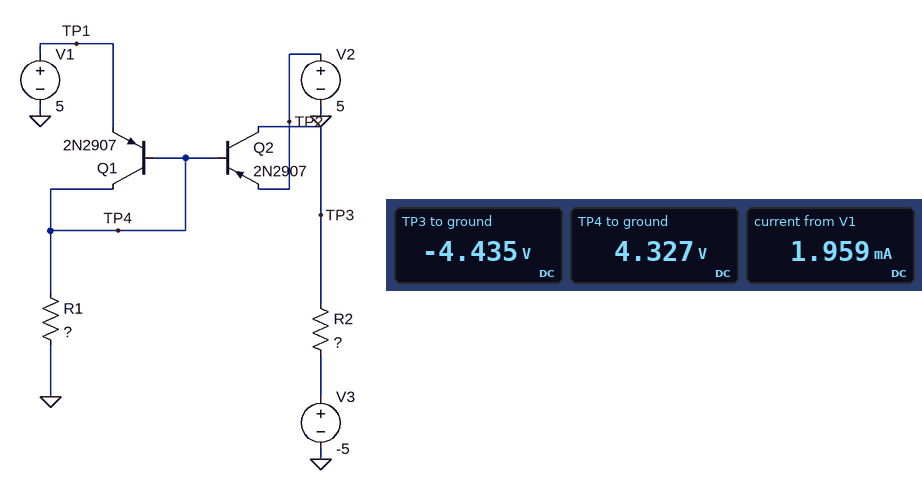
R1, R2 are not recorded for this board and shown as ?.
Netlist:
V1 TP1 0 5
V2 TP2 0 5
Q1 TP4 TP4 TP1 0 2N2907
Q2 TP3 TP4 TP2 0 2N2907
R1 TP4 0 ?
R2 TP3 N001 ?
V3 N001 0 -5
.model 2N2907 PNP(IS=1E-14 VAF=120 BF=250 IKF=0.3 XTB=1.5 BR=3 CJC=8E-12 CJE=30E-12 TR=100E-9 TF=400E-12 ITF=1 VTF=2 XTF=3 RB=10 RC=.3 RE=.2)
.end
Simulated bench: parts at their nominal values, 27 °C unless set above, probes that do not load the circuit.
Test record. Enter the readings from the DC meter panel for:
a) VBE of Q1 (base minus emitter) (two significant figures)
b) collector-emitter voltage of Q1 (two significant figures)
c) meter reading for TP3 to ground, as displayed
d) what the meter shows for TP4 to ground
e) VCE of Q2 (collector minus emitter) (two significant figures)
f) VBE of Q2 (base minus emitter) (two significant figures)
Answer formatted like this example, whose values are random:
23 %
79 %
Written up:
-670 mV
-670 mV
-4.435 V
4.327 V
-9.4 V
-670 mV
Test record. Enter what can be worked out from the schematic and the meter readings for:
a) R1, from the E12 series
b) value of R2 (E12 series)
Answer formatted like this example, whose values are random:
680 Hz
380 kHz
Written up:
2.2 kΩ
270 Ω
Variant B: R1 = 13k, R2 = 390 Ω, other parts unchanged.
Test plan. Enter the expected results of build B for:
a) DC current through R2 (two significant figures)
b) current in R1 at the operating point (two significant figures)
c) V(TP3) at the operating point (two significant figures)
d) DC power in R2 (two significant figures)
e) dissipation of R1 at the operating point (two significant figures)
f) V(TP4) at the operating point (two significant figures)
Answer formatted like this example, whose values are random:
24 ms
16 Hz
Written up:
360 µA
340 µA
-4.9 V
50 µW
1.5 mW
4.4 V
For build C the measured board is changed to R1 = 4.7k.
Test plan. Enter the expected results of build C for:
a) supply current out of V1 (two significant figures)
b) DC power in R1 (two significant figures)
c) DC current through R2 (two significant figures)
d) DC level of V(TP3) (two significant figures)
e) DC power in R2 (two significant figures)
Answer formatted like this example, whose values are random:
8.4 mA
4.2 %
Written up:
920 µA
4.0 mW
990 µA
-4.7 V
260 µW
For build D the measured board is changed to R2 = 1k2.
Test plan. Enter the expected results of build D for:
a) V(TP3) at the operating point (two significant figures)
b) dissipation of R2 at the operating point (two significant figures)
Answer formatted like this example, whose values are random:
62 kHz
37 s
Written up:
-2.5 V
5.1 mW
